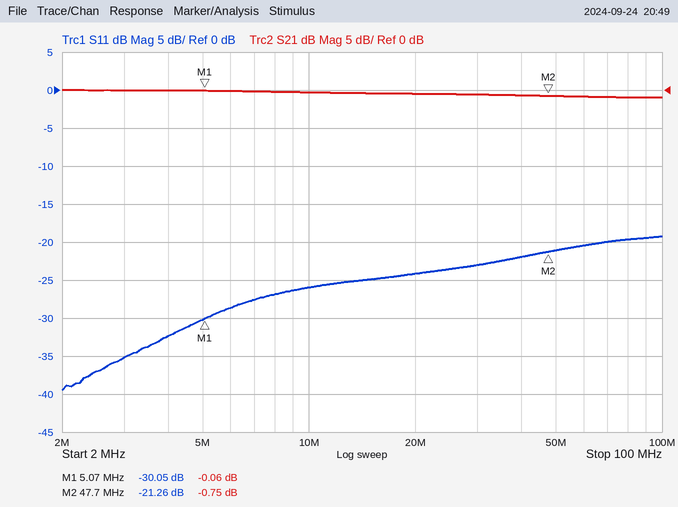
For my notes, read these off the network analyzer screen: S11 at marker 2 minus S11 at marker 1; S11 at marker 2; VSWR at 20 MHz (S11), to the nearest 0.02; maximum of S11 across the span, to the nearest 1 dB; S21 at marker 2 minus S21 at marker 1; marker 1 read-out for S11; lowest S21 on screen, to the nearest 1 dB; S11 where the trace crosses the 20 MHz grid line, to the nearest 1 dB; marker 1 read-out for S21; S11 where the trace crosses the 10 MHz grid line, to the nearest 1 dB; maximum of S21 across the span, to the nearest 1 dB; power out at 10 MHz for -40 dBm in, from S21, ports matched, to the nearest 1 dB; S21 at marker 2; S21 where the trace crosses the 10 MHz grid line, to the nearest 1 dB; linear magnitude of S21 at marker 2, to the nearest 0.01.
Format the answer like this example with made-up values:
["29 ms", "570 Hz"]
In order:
["8.79 dB", "-21.26 dB", "1.14", "-19 dB", "-0.69 dB", "-30.05 dB", "-1 dB", "-24 dB", "-0.06 dB", "-26 dB", "0 dB", "-40 dBm", "-0.75 dB", "0 dB", "0.92"]
